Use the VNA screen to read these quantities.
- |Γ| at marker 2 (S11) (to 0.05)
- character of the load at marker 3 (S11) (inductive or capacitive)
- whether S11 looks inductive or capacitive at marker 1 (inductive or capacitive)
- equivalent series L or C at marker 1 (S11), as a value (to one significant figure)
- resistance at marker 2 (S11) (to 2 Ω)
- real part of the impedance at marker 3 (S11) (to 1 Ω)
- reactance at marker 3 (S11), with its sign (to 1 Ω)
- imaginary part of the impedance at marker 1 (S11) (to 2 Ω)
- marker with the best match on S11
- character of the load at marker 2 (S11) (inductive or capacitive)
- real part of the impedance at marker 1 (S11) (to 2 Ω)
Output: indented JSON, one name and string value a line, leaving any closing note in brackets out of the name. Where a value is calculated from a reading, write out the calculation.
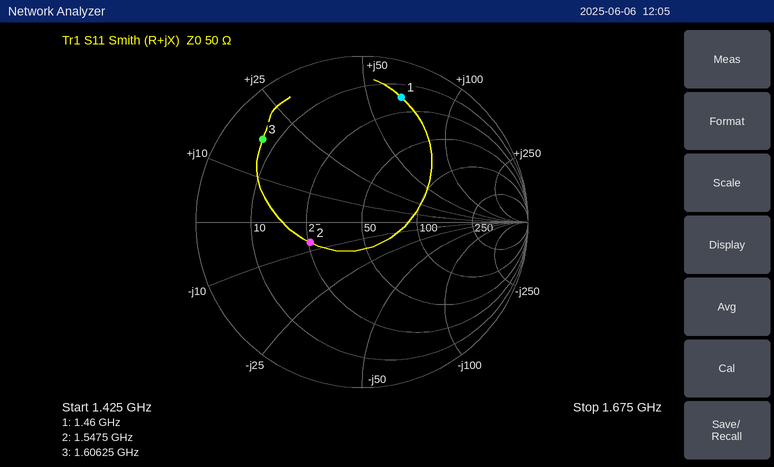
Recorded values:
{
  "|Γ| at marker 2 (S11)": "0.35",
  "character of the load at marker 3 (S11)": "inductive",
  "whether S11 looks inductive or capacitive at marker 1": "inductive",
  "equivalent series L or C at marker 1 (S11), as a value": "L = 66 Ω/(2π × 1.46 GHz) ≈ 7 nH",
  "resistance at marker 2 (S11)": "26 Ω",
  "real part of the impedance at marker 3 (S11)": "7 Ω",
  "reactance at marker 3 (S11), with its sign": "+18 Ω",
  "imaginary part of the impedance at marker 1 (S11)": "+66 Ω",
  "marker with the best match on S11": "marker 2",
  "character of the load at marker 2 (S11)": "capacitive",
  "real part of the impedance at marker 1 (S11)": "16 Ω"
}
